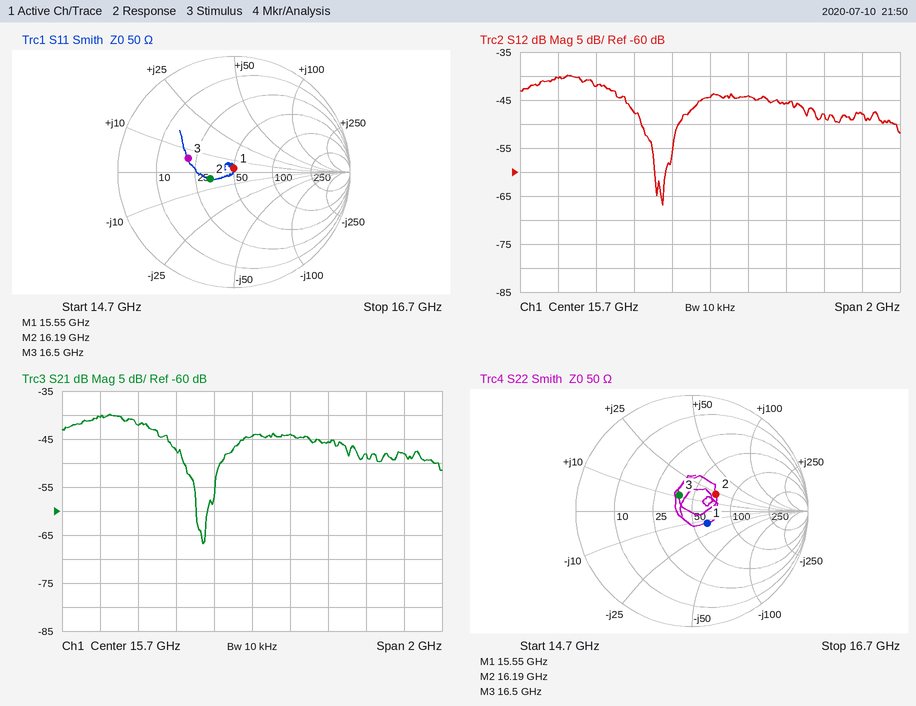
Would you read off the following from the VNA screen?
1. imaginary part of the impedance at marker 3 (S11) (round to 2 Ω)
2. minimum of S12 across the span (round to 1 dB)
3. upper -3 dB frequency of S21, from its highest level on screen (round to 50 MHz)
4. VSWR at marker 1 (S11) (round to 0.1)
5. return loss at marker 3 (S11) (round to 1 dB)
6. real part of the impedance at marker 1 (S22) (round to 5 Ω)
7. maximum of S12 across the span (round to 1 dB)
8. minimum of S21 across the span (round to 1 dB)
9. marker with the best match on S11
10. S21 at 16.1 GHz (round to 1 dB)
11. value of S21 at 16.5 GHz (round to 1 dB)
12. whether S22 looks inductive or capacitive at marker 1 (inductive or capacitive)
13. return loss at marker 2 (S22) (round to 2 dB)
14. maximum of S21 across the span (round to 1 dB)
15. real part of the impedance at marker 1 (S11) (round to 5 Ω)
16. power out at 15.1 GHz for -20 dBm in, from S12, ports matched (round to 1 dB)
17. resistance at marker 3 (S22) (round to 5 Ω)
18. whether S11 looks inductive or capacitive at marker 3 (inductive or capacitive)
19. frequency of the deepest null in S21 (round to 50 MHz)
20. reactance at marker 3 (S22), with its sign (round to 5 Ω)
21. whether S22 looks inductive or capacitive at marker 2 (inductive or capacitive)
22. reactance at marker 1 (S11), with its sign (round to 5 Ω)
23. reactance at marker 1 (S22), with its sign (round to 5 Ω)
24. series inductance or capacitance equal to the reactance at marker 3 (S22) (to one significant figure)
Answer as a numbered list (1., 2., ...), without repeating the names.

1. +6 Ω
2. -67 dB
3. 15.15 GHz
4. 1.1
5. 8 dB
6. 65 Ω
7. -40 dB
8. -67 dB
9. marker 1
10. -46 dB
11. -48 dB
12. capacitive
13. 12 dB
14. -40 dB
15. 50 Ω
16. -62 dBm
17. 40 Ω
18. inductive
19. 15.45 GHz
20. +10 Ω
21. inductive
22. +5 Ω
23. -15 Ω
24. 100 pH
